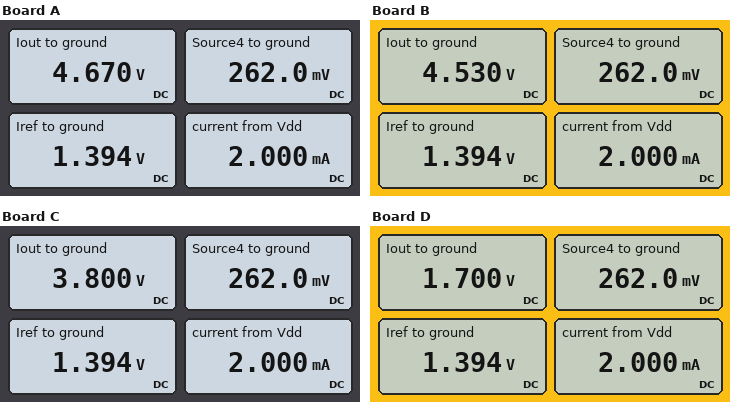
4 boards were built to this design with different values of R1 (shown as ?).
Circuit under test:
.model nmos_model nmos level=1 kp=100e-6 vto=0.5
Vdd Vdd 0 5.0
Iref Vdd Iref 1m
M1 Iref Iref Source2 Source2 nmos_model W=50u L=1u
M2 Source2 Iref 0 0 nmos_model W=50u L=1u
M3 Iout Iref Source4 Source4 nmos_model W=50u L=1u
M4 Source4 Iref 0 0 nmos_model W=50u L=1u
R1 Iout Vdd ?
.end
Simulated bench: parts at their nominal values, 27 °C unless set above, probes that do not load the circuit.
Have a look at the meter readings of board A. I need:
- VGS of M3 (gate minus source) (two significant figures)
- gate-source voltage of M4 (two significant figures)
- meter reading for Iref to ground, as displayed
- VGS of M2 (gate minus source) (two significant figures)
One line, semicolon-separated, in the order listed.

1.1 V; 1.4 V; 1.394 V; 1.4 V
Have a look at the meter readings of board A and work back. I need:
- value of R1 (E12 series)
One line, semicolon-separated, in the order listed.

330 Ω
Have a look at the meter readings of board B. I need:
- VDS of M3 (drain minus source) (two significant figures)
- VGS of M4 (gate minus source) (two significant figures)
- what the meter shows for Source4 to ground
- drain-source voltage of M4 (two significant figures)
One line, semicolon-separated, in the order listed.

4.3 V; 1.4 V; 262.0 mV; 260 mV
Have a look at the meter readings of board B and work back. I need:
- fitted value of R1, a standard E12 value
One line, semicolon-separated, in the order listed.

470 Ω
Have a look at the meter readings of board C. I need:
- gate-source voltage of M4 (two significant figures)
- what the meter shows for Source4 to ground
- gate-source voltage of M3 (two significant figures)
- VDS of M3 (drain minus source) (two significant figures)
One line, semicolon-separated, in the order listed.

1.4 V; 262.0 mV; 1.1 V; 3.5 V
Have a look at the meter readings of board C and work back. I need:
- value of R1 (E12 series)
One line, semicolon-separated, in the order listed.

1.2 kΩ
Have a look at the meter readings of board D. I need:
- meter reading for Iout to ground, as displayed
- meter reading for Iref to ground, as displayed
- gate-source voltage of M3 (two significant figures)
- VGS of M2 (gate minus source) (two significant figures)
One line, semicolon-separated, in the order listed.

1.700 V; 1.394 V; 1.1 V; 1.4 V
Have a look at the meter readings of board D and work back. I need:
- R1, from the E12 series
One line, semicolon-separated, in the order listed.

3.3 kΩ
